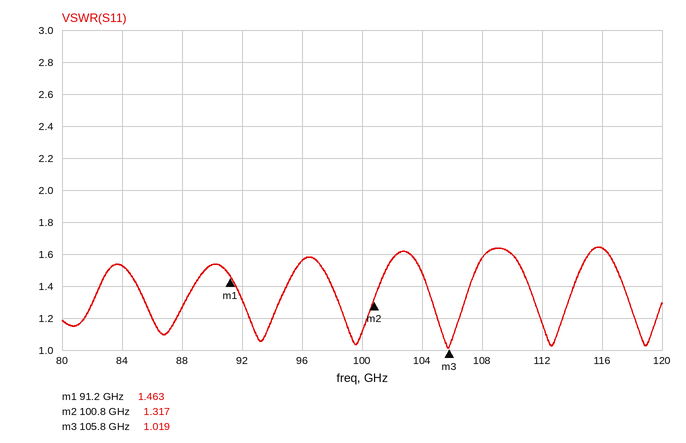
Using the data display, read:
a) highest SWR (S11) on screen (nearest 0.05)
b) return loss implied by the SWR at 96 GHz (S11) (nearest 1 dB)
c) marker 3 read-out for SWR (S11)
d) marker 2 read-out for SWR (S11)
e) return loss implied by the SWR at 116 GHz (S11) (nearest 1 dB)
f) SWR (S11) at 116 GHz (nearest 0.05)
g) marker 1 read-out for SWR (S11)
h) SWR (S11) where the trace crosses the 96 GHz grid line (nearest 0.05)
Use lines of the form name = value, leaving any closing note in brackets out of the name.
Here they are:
highest SWR (S11) on screen = 1.65
return loss implied by the SWR at 96 GHz (S11) = 13 dB
marker 3 read-out for SWR = 1.019
marker 2 read-out for SWR = 1.317
return loss implied by the SWR at 116 GHz (S11) = 12 dB
SWR (S11) at 116 GHz = 1.65
marker 1 read-out for SWR = 1.463
SWR (S11) where the trace crosses the 96 GHz grid line = 1.55
